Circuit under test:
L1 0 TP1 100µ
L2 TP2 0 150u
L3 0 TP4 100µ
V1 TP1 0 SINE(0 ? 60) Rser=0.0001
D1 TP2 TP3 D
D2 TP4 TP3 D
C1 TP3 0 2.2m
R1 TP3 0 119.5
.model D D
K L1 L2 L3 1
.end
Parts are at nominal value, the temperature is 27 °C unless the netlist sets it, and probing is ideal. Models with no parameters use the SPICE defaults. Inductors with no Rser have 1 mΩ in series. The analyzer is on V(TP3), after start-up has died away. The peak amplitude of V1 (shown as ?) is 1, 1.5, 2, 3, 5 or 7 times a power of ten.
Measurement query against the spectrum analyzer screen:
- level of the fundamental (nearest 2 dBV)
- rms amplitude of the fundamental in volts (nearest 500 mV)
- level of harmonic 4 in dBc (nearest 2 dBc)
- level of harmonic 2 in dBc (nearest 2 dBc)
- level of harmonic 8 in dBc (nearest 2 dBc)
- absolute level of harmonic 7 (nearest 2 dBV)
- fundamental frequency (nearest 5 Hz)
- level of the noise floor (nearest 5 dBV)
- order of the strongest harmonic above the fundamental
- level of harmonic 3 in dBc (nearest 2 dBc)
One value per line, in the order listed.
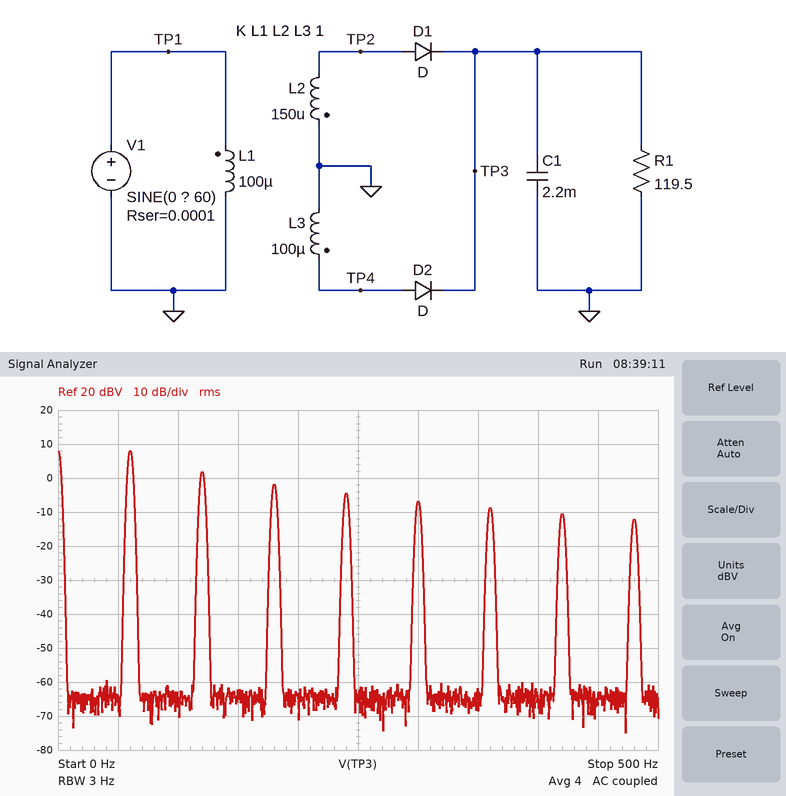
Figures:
8 dBV
2.5 V
-12 dBc
-6 dBc
-20 dBc
-10 dBV
60 Hz
-65 dBV
2
-10 dBc
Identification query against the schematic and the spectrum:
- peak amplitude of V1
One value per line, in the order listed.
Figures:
150 V
